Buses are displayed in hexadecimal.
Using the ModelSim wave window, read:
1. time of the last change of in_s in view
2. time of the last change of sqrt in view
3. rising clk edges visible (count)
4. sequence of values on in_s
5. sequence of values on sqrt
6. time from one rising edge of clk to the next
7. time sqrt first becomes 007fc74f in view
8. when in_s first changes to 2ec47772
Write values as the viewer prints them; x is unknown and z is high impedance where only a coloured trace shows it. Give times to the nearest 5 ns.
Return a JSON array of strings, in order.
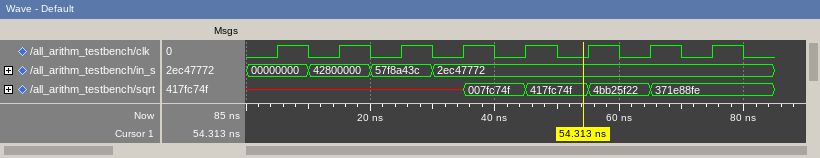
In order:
["30 ns", "65 ns", "8", "00000000, 42800000, 57f8a43c, 2ec47772", "x, 007fc74f, 417fc74f, 4bb25f22, 371e88fe", "10 ns", "35 ns", "30 ns"]
